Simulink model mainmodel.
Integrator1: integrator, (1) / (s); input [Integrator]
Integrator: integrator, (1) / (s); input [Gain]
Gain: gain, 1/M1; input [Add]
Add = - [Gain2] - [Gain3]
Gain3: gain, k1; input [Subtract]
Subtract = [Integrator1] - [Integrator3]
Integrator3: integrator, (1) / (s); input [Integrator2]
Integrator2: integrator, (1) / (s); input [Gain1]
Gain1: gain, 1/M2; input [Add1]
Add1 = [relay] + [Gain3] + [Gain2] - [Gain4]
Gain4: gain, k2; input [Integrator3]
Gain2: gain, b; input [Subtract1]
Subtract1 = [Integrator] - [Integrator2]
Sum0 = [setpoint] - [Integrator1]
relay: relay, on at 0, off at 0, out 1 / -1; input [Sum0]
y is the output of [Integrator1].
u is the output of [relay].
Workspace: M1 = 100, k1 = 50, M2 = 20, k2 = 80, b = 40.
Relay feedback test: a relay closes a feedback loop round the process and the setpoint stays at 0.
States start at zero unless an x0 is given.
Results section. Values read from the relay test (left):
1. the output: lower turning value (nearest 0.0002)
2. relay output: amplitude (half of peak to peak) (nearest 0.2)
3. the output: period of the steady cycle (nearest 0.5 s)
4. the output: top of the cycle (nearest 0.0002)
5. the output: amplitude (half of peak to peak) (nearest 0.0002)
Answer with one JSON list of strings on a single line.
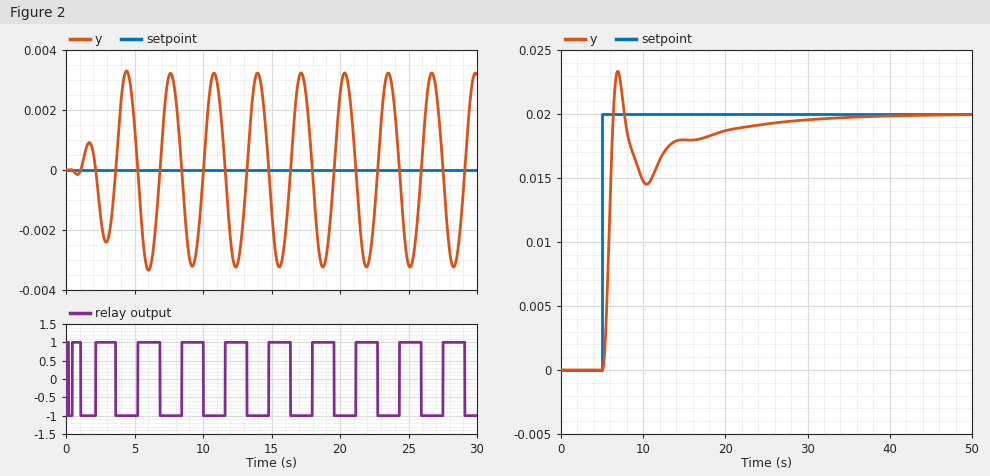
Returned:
["-0.0032", "1.0", "3.0 s", "0.0032", "0.0032"]
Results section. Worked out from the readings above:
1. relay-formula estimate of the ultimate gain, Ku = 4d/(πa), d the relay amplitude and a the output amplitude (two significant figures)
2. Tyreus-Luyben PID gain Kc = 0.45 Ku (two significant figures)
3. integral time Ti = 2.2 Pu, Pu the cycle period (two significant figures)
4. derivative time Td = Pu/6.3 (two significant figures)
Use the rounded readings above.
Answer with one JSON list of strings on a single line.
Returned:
["400", "180", "6.6 s", "0.48 s"]
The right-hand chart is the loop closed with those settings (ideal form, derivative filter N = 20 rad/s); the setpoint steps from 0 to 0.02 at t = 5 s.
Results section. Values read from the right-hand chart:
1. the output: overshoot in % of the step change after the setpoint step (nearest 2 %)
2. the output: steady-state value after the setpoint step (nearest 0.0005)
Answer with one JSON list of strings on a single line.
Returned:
["16 %", "0.0200"]
